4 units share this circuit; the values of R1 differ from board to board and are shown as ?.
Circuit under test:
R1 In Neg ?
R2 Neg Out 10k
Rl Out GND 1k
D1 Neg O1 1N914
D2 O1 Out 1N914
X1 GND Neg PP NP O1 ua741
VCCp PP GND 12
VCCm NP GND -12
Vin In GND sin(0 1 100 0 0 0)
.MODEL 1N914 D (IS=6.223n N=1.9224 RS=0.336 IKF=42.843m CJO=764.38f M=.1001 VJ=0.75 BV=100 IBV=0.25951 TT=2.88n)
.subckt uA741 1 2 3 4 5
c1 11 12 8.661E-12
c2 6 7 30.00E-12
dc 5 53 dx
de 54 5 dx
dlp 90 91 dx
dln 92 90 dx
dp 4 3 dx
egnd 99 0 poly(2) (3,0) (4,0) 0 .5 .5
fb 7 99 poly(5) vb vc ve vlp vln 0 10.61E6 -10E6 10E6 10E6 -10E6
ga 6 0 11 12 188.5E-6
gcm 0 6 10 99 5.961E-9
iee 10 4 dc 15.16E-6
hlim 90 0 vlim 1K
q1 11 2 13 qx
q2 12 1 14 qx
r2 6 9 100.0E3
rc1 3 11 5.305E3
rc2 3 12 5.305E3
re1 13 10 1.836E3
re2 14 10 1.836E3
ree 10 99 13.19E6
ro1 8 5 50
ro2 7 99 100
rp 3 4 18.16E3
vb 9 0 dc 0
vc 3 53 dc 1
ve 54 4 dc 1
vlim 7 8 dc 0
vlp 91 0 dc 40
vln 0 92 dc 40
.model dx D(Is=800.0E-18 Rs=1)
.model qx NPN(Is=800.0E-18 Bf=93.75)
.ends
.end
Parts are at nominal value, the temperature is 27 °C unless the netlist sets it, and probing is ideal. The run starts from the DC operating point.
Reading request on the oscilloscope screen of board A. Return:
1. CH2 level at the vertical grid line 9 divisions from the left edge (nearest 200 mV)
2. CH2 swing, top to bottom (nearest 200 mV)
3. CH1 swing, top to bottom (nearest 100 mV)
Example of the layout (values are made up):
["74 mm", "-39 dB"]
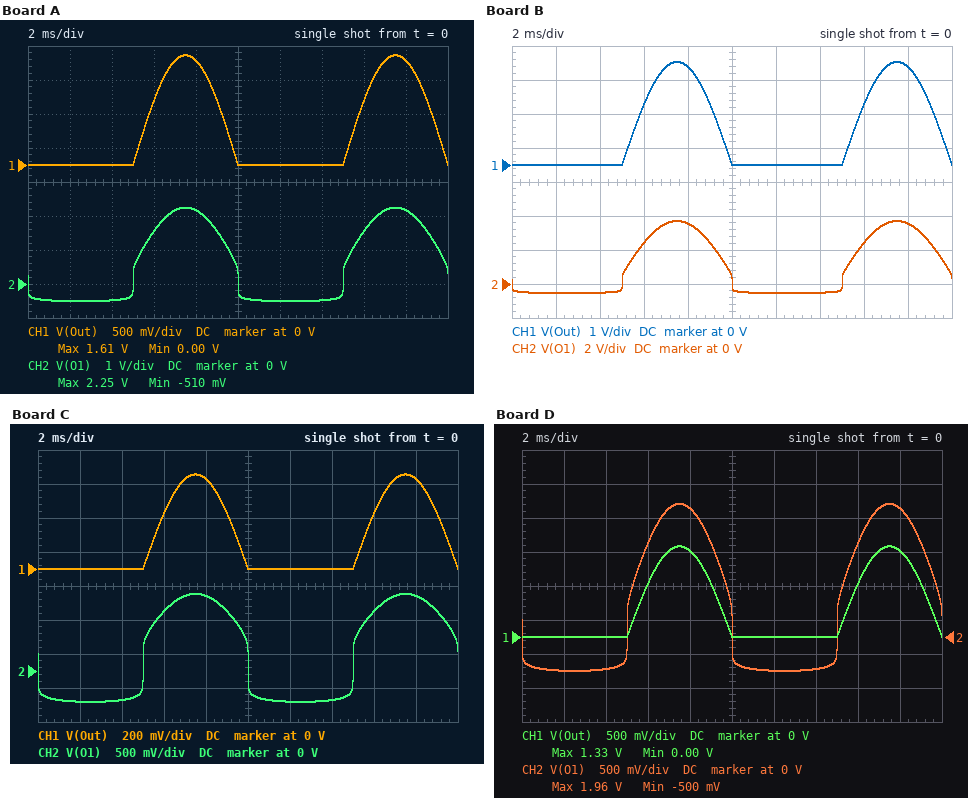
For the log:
["2.2 V", "2.8 V", "1.6 V"]
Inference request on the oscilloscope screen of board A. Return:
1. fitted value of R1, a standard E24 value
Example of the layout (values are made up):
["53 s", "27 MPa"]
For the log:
["6.2 kΩ"]
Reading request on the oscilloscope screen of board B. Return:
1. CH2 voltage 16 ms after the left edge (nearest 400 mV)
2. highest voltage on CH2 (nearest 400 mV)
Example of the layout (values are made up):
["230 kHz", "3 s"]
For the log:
["2.4 V", "3.6 V"]
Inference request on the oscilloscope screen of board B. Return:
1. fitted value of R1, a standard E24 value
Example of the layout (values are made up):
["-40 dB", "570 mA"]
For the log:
["3.3 kΩ"]
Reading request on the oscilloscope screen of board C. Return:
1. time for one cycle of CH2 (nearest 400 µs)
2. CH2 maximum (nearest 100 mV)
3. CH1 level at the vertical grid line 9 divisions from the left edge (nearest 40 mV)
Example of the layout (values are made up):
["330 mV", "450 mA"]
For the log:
["10.0 ms", "1.1 V", "520 mV"]
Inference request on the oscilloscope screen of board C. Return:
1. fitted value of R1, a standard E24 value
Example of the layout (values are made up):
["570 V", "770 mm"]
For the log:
["18 kΩ"]
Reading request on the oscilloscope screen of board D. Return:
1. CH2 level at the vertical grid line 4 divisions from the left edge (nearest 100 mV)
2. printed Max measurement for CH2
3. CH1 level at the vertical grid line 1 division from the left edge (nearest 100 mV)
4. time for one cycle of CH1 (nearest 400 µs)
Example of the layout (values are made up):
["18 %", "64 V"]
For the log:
["1.9 V", "1.96 V", "0 V", "10.0 ms"]
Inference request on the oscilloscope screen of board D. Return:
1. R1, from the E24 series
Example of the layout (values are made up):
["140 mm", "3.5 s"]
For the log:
["7.5 kΩ"]
